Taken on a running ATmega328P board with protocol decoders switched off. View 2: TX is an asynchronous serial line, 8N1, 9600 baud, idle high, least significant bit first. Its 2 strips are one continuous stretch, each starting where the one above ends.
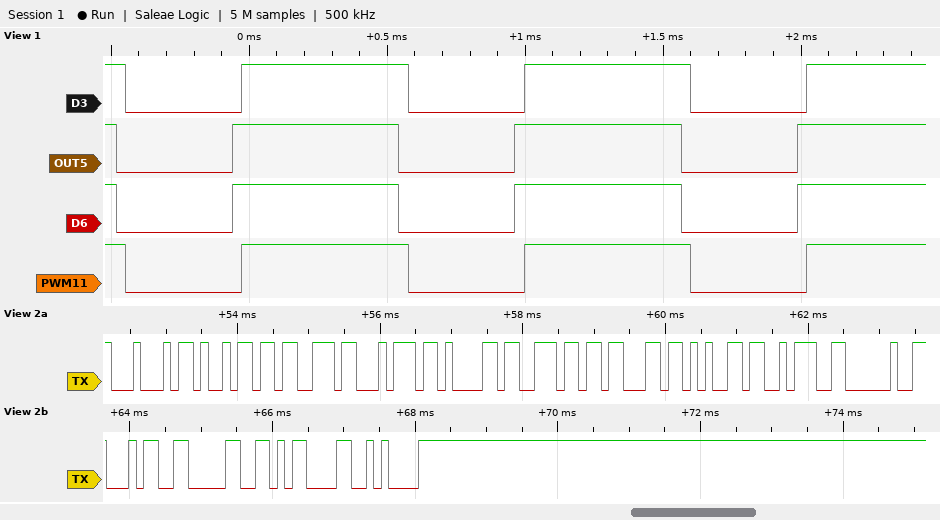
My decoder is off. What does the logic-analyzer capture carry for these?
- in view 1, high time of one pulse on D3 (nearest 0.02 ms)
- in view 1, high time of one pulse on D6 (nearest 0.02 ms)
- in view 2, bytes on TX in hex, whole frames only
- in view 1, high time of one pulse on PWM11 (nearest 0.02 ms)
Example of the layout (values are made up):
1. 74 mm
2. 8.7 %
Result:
1. 0.60 ms
2. 0.60 ms
3. 44 69 73 74 61 6E 63 65 3A 20 34 30 0D 0A
4. 0.60 ms
